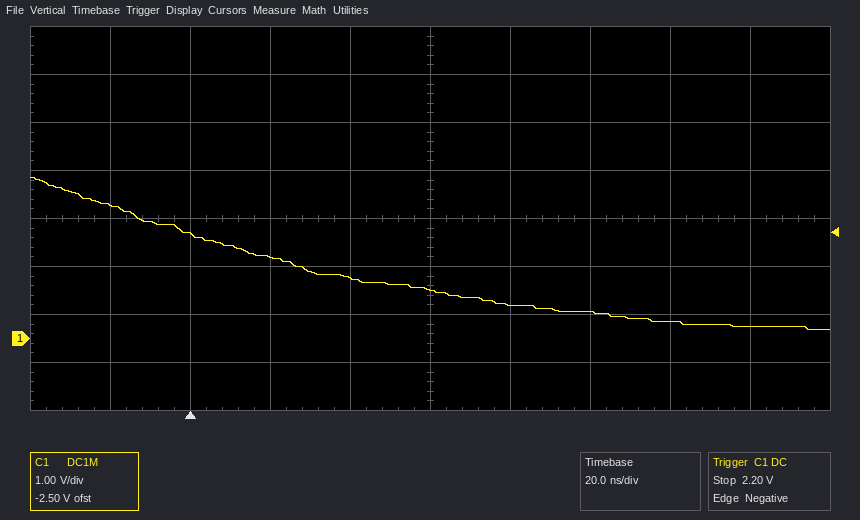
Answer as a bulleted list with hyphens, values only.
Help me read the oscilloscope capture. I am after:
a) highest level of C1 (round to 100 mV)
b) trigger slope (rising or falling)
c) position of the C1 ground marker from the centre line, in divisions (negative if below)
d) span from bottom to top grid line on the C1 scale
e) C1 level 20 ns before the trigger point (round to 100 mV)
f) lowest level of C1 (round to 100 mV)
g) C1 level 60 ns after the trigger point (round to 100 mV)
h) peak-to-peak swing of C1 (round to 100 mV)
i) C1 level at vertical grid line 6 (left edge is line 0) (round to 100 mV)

- 3.4 V
- falling
- -2.5 div
- 8 V
- 2.8 V
- 200 mV
- 1.0 V
- 3.2 V
- 700 mV
